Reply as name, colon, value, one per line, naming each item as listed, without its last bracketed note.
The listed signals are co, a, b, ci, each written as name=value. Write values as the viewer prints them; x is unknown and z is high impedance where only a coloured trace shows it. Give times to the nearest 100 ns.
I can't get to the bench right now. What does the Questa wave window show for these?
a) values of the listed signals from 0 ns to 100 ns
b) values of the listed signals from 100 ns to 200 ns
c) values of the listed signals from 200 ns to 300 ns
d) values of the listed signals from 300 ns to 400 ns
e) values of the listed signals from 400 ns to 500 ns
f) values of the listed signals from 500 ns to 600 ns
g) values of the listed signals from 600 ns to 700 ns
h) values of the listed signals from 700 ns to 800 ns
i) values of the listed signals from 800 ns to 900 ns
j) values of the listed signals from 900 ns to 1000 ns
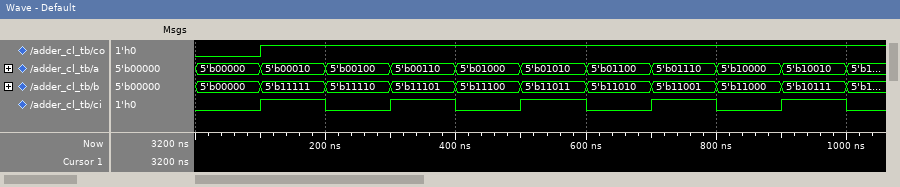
values of the listed signals from 0 ns to 100 ns: co=0, a=5'b00000, b=5'b00000, ci=0
values of the listed signals from 100 ns to 200 ns: co=1, a=5'b00010, b=5'b11111, ci=1
values of the listed signals from 200 ns to 300 ns: co=1, a=5'b00100, b=5'b11110, ci=0
values of the listed signals from 300 ns to 400 ns: co=1, a=5'b00110, b=5'b11101, ci=1
values of the listed signals from 400 ns to 500 ns: co=1, a=5'b01000, b=5'b11100, ci=0
values of the listed signals from 500 ns to 600 ns: co=1, a=5'b01010, b=5'b11011, ci=1
values of the listed signals from 600 ns to 700 ns: co=1, a=5'b01100, b=5'b11010, ci=0
values of the listed signals from 700 ns to 800 ns: co=1, a=5'b01110, b=5'b11001, ci=1
values of the listed signals from 800 ns to 900 ns: co=1, a=5'b10000, b=5'b11000, ci=0
values of the listed signals from 900 ns to 1000 ns: co=1, a=5'b10010, b=5'b10111, ci=1
